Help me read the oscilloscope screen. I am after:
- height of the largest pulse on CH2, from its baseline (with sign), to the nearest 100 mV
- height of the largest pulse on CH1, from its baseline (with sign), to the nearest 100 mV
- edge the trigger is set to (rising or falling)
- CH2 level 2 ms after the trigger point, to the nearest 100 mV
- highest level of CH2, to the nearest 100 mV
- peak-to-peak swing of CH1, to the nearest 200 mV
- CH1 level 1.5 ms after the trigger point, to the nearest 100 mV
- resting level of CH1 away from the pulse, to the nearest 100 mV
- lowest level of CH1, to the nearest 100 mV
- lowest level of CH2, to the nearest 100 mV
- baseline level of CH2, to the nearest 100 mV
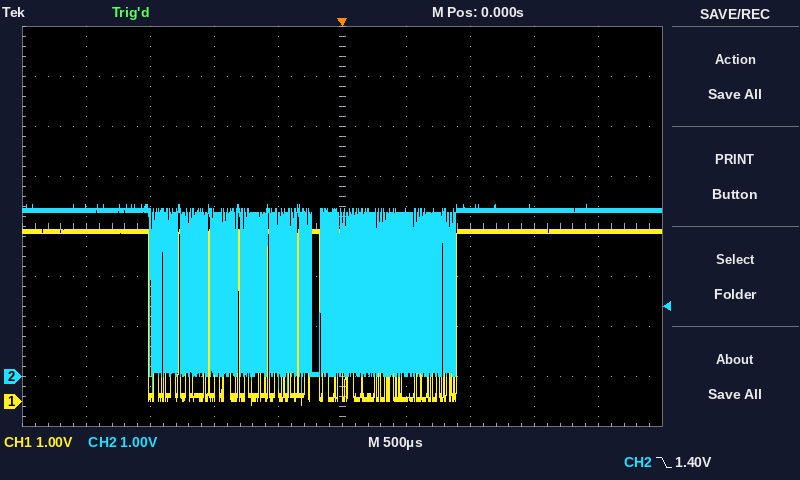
-3.6 V
-3.5 V
falling
3.3 V
3.4 V
3.6 V
3.4 V
3.4 V
-100 mV
-300 mV
3.3 V
